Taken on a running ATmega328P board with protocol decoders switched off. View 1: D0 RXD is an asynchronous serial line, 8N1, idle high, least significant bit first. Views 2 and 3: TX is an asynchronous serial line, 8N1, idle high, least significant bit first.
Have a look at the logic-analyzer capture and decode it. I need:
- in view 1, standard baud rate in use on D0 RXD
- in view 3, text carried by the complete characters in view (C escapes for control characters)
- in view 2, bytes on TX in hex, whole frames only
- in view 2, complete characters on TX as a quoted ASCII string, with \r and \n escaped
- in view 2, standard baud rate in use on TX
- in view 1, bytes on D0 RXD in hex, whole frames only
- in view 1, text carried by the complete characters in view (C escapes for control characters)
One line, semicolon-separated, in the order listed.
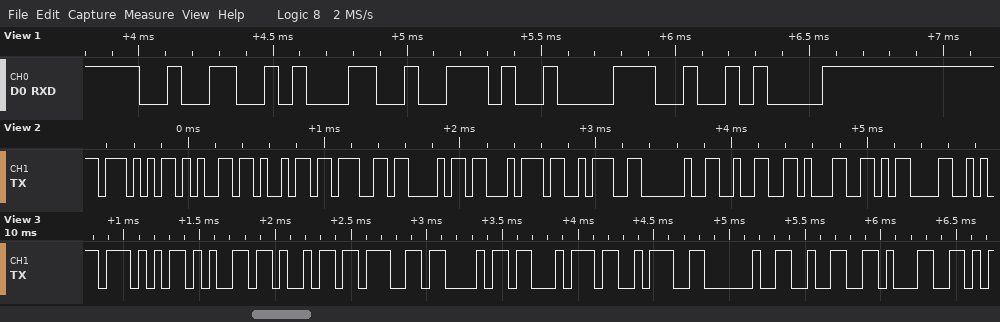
19200 baud; "Weight: 21"; 57 65 69 67 68 74 3A 20 32 31 0D; "Weight: 21\r"; 19200 baud; 32 31 2E 38 0A; "21.8\n"
